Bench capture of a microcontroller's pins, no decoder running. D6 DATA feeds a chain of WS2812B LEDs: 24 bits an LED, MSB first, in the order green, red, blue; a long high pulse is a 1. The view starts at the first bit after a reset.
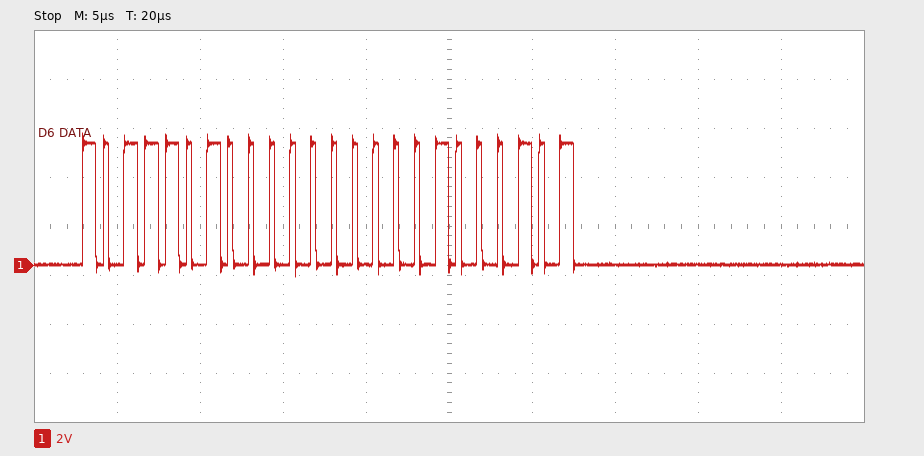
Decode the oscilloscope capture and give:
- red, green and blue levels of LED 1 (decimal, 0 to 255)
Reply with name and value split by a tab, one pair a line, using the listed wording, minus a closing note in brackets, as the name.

red, green and blue levels of LED 1	0, 186, 69
